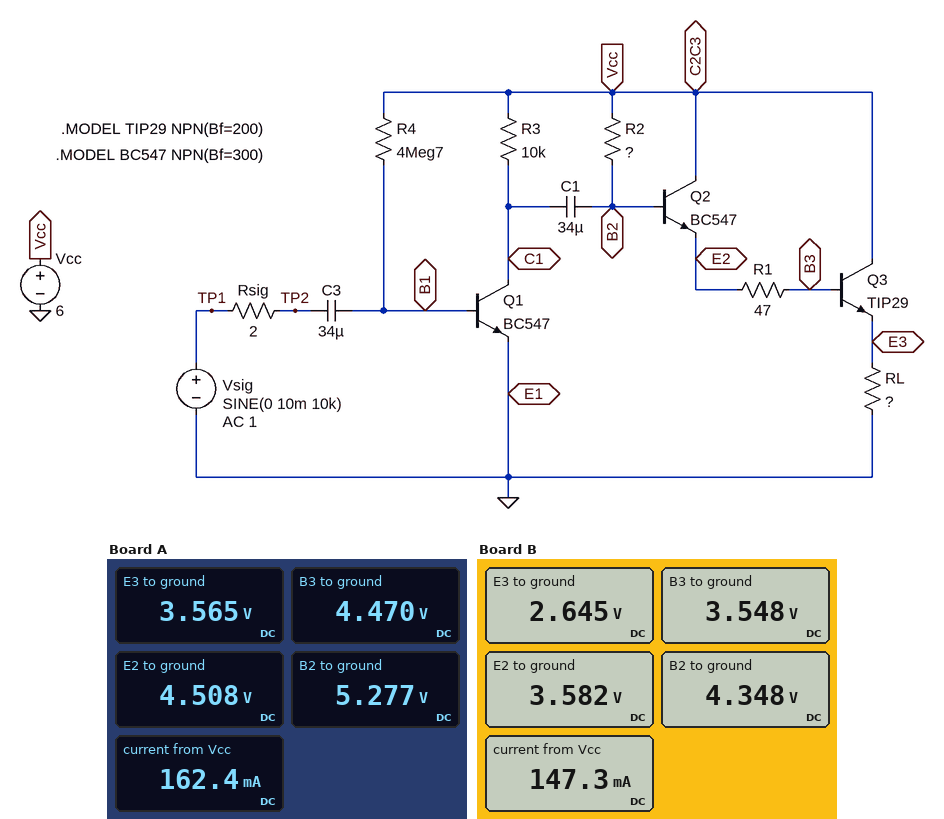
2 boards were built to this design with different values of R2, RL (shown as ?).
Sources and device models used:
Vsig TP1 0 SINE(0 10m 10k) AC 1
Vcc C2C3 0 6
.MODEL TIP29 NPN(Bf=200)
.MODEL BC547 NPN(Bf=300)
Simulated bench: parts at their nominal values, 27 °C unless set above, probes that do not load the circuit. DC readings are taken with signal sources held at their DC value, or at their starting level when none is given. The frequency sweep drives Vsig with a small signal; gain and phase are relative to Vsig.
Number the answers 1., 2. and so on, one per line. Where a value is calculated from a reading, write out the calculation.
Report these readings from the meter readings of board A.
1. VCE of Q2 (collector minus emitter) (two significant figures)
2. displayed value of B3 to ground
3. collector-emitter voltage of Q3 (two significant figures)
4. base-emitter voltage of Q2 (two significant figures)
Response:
1. 6 V - 4.508 V = 1.5 V
2. 4.470 V
3. 6 V - 3.565 V = 2.4 V
4. 5.277 V - 4.508 V = 770 mV
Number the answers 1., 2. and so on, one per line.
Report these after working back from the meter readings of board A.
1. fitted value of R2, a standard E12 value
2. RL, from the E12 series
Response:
1. 270 kΩ
2. 22 Ω
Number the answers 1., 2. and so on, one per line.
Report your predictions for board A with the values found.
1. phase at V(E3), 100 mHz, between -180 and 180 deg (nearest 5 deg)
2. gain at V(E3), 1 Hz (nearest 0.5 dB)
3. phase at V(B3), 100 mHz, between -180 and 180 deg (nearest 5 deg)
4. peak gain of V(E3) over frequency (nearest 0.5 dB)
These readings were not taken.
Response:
1. -105 deg
2. 41.5 dB
3. -105 deg
4. 41.5 dB
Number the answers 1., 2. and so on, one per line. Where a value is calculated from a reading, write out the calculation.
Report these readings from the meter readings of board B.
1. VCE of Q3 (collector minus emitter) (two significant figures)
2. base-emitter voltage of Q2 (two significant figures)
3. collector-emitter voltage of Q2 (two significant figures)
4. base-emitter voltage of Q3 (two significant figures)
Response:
1. 6 V - 2.645 V = 3.4 V
2. 4.348 V - 3.582 V = 770 mV
3. 6 V - 3.582 V = 2.4 V
4. 3.548 V - 2.645 V = 900 mV
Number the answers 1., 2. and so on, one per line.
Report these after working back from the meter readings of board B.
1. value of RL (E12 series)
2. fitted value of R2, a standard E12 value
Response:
1. 18 Ω
2. 680 kΩ
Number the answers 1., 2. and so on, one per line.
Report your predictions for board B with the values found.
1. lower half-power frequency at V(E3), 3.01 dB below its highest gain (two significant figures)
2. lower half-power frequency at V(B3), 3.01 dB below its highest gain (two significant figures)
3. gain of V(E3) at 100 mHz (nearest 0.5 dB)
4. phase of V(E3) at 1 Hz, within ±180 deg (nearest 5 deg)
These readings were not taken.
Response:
1. 200 mHz
2. 200 mHz
3. 34.5 dB
4. -170 deg
